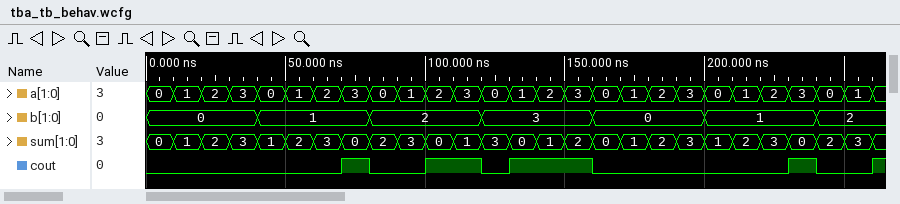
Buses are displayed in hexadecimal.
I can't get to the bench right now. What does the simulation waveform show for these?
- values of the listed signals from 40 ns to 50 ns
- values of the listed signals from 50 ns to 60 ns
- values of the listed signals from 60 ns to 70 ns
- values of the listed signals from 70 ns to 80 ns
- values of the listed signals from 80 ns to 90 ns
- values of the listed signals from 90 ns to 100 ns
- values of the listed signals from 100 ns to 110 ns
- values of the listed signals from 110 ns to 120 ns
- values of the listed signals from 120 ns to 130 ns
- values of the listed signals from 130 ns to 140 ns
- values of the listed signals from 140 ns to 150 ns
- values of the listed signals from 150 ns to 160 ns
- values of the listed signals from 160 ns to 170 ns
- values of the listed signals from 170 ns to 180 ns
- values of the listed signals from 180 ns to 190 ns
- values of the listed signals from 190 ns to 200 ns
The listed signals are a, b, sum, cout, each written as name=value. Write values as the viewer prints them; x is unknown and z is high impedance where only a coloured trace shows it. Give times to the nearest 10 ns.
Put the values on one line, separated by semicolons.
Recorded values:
a=0, b=1, sum=1, cout=0; a=1, b=1, sum=2, cout=0; a=2, b=1, sum=3, cout=0; a=3, b=1, sum=0, cout=1; a=0, b=2, sum=2, cout=0; a=1, b=2, sum=3, cout=0; a=2, b=2, sum=0, cout=1; a=3, b=2, sum=1, cout=1; a=0, b=3, sum=3, cout=0; a=1, b=3, sum=0, cout=1; a=2, b=3, sum=1, cout=1; a=3, b=3, sum=2, cout=1; a=0, b=0, sum=0, cout=0; a=1, b=0, sum=1, cout=0; a=2, b=0, sum=2, cout=0; a=3, b=0, sum=3, cout=0
